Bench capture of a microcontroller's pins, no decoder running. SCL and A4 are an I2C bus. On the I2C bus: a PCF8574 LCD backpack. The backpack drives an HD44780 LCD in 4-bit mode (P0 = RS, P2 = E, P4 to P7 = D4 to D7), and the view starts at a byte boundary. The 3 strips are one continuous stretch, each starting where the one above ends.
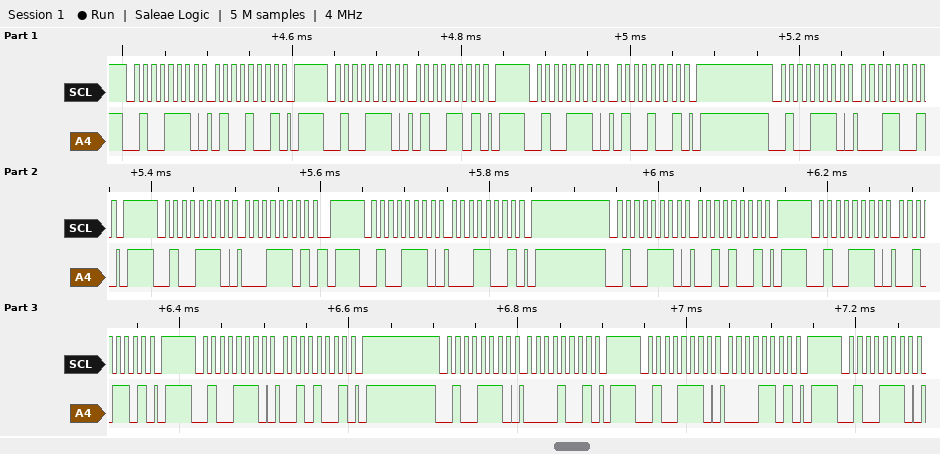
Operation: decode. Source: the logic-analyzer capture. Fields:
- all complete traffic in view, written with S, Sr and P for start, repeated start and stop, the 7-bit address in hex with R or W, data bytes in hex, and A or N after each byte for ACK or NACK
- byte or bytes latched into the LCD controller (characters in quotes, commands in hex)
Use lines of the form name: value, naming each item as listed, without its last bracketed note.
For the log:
all complete traffic in view, written with S, Sr and P for start, repeated start and stop, the 7-bit address in hex with R or W, data bytes in hex, and A or N after each byte for ACK or NACK: S 27W A 49 A P S 27W A 4D A P S 27W A 49 A P S 27W A 19 A P S 27W A 1D A P S 27W A 19 A P S 27W A 29 A P S 27W A 2D A P S 27W A 29 A P S 27W A 09 A P S 27W A 0D A P S 27W A
byte or bytes latched into the LCD controller: 'A'
